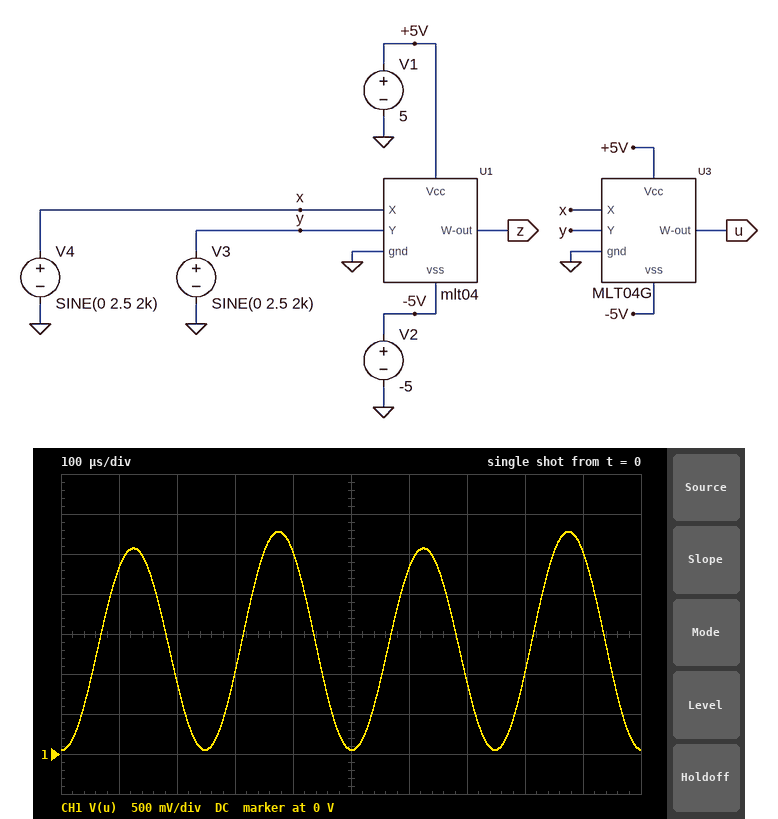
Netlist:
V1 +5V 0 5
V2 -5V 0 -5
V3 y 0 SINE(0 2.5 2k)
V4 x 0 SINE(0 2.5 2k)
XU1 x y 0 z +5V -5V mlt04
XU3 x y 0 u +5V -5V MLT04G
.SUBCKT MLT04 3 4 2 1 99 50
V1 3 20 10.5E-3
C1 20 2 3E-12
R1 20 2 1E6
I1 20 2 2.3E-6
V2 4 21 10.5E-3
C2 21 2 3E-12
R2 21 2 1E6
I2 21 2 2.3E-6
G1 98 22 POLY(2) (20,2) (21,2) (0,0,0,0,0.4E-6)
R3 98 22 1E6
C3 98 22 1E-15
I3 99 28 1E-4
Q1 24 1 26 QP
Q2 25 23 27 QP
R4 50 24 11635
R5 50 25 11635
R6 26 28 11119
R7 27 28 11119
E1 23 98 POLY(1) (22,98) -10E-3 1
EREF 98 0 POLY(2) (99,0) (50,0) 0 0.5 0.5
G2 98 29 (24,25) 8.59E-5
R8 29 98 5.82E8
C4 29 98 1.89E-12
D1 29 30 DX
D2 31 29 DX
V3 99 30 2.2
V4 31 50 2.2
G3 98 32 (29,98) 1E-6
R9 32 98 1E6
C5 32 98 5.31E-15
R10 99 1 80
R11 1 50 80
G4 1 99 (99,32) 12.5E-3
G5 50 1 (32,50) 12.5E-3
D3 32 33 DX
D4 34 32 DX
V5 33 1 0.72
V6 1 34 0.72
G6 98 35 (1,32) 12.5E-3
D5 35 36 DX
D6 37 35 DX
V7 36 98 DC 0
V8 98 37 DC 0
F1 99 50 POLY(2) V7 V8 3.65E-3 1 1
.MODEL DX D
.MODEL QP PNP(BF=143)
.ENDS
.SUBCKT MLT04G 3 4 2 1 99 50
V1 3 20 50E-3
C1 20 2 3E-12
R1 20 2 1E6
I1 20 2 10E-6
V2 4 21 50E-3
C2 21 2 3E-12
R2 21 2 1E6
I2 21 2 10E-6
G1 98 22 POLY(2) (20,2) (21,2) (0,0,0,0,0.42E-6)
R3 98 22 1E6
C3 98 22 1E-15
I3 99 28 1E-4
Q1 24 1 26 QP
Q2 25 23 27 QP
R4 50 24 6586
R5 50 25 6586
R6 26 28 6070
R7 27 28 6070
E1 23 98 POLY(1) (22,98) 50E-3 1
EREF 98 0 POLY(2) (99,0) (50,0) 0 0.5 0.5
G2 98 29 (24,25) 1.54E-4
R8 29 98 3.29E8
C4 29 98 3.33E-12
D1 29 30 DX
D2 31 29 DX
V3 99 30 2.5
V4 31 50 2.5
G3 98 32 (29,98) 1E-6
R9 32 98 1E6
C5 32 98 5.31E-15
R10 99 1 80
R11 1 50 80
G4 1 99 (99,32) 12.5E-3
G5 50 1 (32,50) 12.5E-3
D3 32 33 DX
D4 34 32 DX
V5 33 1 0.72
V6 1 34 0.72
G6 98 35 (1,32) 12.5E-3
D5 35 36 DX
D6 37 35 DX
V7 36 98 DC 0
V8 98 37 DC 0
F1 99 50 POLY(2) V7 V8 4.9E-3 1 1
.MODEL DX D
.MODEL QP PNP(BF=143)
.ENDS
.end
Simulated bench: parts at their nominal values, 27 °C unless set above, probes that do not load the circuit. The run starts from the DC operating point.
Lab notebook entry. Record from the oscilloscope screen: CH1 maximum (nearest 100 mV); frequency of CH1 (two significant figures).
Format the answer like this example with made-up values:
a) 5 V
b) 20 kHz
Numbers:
a) 2.8 V
b) 4.0 kHz
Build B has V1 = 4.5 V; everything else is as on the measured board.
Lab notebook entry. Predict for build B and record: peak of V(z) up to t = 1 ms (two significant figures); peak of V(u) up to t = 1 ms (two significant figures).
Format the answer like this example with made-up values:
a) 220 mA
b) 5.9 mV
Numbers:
a) 2.3 V
b) 2.5 V
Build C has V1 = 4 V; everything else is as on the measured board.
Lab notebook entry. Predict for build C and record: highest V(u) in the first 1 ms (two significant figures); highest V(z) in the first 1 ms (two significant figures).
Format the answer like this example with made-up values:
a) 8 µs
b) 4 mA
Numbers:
a) 2.1 V
b) 2.0 V
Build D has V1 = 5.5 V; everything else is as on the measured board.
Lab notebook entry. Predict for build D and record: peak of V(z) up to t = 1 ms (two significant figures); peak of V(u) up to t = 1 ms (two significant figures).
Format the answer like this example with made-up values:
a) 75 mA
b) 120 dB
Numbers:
a) 2.8 V
b) 3.0 V
